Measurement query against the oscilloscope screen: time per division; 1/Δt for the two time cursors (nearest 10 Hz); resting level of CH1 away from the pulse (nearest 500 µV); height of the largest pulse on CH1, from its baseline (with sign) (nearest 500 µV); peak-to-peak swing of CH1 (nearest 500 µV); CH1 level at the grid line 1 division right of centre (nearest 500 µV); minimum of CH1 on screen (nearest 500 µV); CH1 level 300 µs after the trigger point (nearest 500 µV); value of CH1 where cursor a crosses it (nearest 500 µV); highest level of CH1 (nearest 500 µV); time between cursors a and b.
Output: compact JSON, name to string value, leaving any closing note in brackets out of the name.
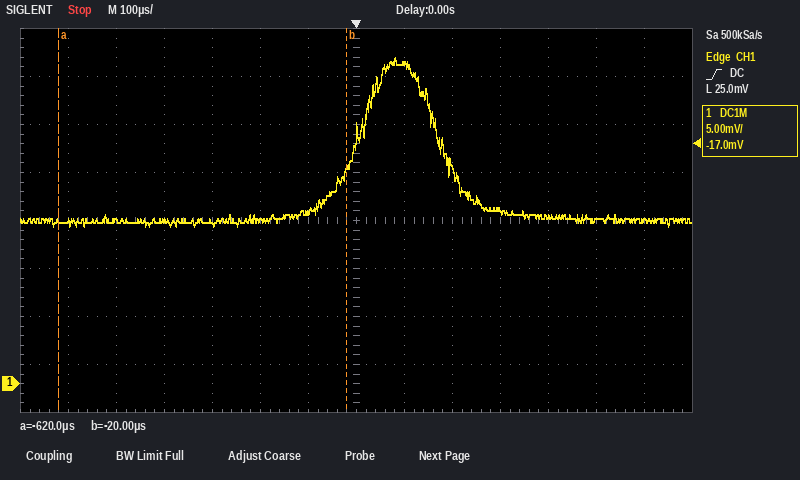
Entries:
{"time per division": "100 µs", "1/Δt for the two time cursors": "1.67 kHz", "resting level of CH1 away from the pulse": "17.0 mV", "height of the largest pulse on CH1, from its baseline (with sign)": "+17.0 mV", "peak-to-peak swing of CH1": "17.5 mV", "CH1 level at the grid line 1 division right of centre": "33.5 mV", "minimum of CH1 on screen": "16.5 mV", "CH1 level 300 µs after the trigger point": "18.0 mV", "value of CH1 where cursor a crosses it": "17.0 mV", "highest level of CH1": "34.0 mV", "time between cursors a and b": "600 µs"}
